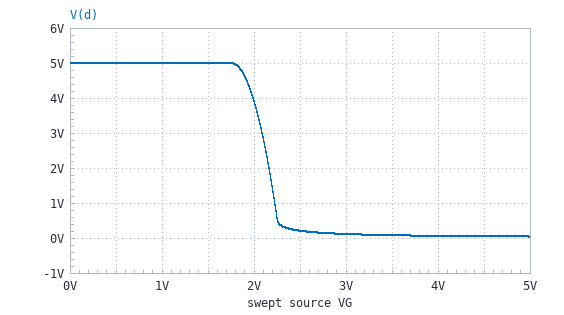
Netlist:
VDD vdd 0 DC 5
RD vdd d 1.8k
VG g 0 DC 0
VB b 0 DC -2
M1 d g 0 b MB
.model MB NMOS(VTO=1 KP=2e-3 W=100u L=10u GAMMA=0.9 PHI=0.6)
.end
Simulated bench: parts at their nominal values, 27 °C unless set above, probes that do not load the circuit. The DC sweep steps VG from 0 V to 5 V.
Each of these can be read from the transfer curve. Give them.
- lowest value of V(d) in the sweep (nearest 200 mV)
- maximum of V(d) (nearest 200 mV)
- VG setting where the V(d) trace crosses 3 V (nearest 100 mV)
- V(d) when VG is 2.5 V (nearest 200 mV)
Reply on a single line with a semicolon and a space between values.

0 V; 5.0 V; 2.1 V; 200 mV
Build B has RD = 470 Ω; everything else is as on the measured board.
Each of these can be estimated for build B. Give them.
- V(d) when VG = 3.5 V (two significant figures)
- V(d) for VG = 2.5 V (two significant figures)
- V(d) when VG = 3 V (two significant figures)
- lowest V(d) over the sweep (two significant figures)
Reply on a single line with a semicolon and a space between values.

310 mV; 2.4 V; 480 mV; 160 mV
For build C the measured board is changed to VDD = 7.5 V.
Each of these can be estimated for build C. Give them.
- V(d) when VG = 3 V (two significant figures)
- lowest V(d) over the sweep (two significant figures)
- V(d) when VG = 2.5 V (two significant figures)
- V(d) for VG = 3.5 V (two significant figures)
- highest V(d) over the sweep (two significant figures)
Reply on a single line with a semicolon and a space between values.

180 mV; 64 mV; 350 mV; 120 mV; 7.5 V
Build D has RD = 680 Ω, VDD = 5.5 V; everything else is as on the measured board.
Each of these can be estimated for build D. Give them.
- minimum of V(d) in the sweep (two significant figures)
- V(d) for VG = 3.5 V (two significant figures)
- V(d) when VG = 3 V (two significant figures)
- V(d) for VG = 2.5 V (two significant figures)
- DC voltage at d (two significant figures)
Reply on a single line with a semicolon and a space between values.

120 mV; 240 mV; 350 mV; 1.7 V; 5.5 V
